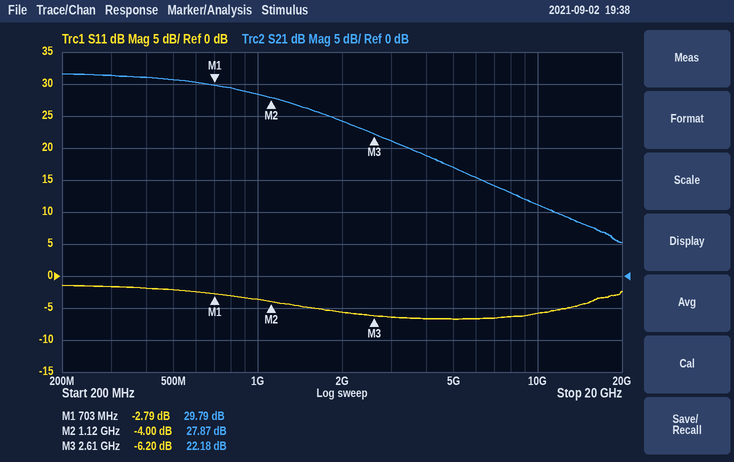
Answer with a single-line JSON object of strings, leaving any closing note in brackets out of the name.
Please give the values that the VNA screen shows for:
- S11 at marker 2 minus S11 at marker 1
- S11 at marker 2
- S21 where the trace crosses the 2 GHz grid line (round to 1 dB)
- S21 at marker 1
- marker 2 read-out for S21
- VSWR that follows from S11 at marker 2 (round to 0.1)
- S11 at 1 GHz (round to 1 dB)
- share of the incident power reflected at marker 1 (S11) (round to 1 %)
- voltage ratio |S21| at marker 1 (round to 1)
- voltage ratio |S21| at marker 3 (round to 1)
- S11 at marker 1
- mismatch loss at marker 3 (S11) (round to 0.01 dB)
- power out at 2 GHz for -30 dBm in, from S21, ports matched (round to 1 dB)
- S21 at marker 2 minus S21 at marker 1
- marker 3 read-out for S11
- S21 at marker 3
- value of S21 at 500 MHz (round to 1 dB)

{"S11 at marker 2 minus S11 at marker 1": "-1.21 dB", "S11 at marker 2": "-4.00 dB", "S21 where the trace crosses the 2 GHz grid line": "24 dB", "S21 at marker 1": "29.79 dB", "marker 2 read-out for S21": "27.87 dB", "VSWR that follows from S11 at marker 2": "4.4", "S11 at 1 GHz": "-4 dB", "share of the incident power reflected at marker 1 (S11)": "53 %", "voltage ratio |S21| at marker 1": "31", "voltage ratio |S21| at marker 3": "13", "S11 at marker 1": "-2.79 dB", "mismatch loss at marker 3 (S11)": "1.19 dB", "power out at 2 GHz for -30 dBm in, from S21, ports matched": "-6 dBm", "S21 at marker 2 minus S21 at marker 1": "-1.92 dB", "marker 3 read-out for S11": "-6.20 dB", "S21 at marker 3": "22.18 dB", "value of S21 at 500 MHz": "31 dB"}
